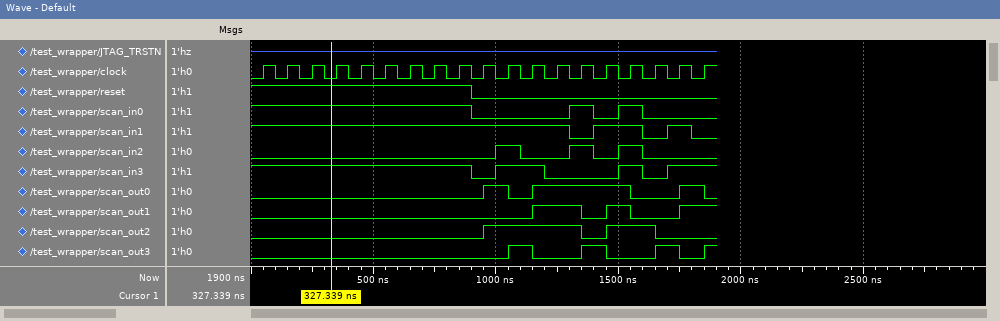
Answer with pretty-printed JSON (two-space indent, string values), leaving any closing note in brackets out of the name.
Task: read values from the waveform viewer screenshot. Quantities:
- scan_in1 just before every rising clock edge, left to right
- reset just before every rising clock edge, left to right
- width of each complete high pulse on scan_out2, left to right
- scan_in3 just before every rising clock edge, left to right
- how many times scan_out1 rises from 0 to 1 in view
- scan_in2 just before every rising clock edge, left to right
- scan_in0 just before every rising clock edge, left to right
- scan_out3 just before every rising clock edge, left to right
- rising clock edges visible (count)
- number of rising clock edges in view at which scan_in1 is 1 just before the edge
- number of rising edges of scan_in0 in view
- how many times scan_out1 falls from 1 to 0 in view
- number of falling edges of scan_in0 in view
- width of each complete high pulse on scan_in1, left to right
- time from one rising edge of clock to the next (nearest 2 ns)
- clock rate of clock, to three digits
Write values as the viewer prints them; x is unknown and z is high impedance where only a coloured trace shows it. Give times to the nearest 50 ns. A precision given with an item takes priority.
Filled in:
{
  "scan_in1 just before every rising clock edge, left to right": "1 1 1 1 1 1 1 1 1 1 1 1 1 0 1 1 0 1 0",
  "reset just before every rising clock edge, left to right": "1 1 1 1 1 1 1 1 1 0 0 0 0 0 0 0 0 0 0",
  "width of each complete high pulse on scan_out2, left to right": "400 ns, 200 ns",
  "scan_in3 just before every rising clock edge, left to right": "1 1 1 1 1 1 1 1 1 0 1 1 0 0 0 1 0 1 1",
  "how many times scan_out1 rises from 0 to 1 in view": "3",
  "scan_in2 just before every rising clock edge, left to right": "0 0 0 0 0 0 0 0 0 0 1 0 0 1 0 1 0 0 0",
  "scan_in0 just before every rising clock edge, left to right": "1 1 1 1 1 1 1 1 1 0 0 0 0 1 0 1 0 0 0",
  "scan_out3 just before every rising clock edge, left to right": "0 0 0 0 0 0 0 0 0 0 0 1 0 0 1 0 0 1 0",
  "rising clock edges visible": "19",
  "number of rising clock edges in view at which scan_in1 is 1 just before the edge": "16",
  "number of rising edges of scan_in0 in view": "2",
  "how many times scan_out1 falls from 1 to 0 in view": "2",
  "number of falling edges of scan_in0 in view": "3",
  "width of each complete high pulse on scan_in1, left to right": "200 ns, 100 ns",
  "time from one rising edge of clock to the next": "100 ns",
  "clock rate of clock, to three digits": "10.0 MHz"
}
